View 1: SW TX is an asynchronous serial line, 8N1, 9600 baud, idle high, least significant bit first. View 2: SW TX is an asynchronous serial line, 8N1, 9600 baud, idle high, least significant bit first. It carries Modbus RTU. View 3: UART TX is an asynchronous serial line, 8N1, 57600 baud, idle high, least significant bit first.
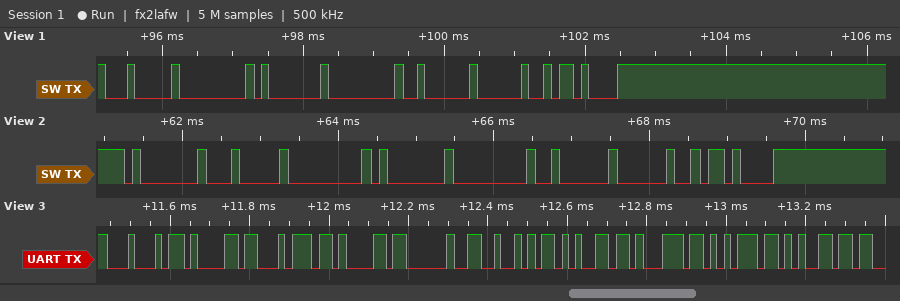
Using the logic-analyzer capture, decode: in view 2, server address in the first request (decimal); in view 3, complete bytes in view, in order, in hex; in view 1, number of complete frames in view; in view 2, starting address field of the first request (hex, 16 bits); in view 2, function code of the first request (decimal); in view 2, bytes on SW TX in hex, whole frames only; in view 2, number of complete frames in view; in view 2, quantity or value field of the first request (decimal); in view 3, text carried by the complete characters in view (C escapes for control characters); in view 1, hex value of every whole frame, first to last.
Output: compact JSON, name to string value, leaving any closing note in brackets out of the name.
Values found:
{"in view 2, server address in the first request": "1", "in view 3, complete bytes in view, in order, in hex": "44 61 74 61 20 52 65 71 75 65", "in view 1, number of complete frames in view": "7", "in view 2, starting address field of the first request": "0x0001", "in view 2, function code of the first request": "4", "in view 2, bytes on SW TX in hex, whole frames only": "0x01 0x04 0x00 0x01 0x00 0x02 0x20 0x0B", "in view 2, number of complete frames in view": "8", "in view 2, quantity or value field of the first request": "2", "in view 3, text carried by the complete characters in view": "\"Data Reque\"", "in view 1, hex value of every whole frame, first to last": "04 00 01 00 02 20 0B"}
